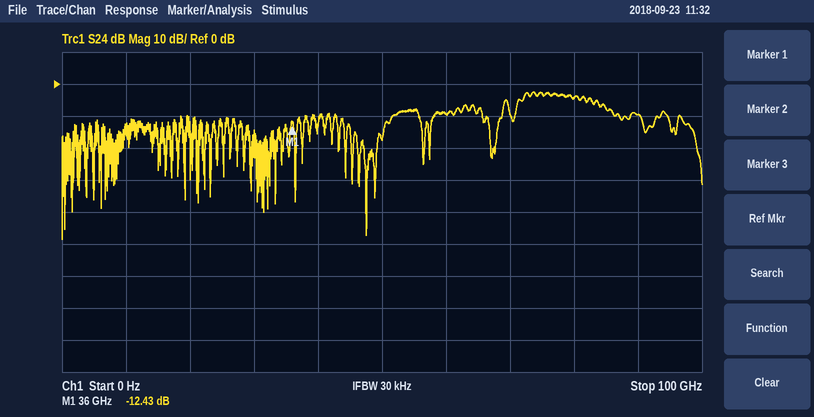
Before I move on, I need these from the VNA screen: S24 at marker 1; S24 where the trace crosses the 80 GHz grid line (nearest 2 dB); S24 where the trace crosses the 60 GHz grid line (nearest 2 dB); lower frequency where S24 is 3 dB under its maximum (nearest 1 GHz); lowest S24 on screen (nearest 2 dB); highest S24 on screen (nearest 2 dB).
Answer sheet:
-12.43 dB
-4 dB
-10 dB
71 GHz
-48 dB
-2 dB
